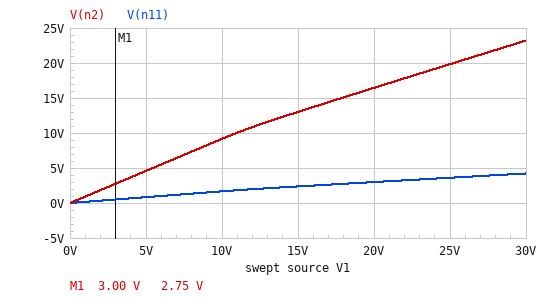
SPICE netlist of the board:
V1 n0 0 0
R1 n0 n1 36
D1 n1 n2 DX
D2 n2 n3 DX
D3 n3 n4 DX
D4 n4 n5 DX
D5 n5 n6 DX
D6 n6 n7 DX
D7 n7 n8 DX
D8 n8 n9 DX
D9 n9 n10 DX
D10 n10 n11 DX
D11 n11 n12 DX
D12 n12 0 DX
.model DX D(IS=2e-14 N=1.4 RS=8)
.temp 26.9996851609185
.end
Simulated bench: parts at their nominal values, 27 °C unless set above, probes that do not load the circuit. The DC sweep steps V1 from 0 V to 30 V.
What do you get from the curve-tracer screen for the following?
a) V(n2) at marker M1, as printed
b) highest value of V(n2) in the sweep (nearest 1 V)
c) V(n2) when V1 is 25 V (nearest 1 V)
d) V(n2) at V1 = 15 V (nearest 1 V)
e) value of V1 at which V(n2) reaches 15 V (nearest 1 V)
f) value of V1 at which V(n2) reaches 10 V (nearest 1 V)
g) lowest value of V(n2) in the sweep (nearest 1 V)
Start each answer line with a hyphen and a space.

- 2.75 V
- 23 V
- 20 V
- 13 V
- 18 V
- 11 V
- 0 V
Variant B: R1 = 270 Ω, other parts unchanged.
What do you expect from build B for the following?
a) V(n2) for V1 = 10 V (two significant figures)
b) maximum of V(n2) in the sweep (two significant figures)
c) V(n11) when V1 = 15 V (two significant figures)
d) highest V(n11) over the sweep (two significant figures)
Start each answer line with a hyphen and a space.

- 9.1 V
- 16 V
- 2.1 V
- 2.8 V
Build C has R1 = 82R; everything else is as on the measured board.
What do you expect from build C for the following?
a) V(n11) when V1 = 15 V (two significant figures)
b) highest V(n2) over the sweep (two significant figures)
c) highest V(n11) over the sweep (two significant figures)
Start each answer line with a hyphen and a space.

- 2.3 V
- 20 V
- 3.7 V
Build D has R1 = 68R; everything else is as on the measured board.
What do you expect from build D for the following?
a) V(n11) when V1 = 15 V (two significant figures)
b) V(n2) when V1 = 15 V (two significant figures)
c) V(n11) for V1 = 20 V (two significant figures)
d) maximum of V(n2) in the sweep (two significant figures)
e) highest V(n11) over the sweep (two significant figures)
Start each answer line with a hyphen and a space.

- 2.3 V
- 13 V
- 2.8 V
- 21 V
- 3.8 V
